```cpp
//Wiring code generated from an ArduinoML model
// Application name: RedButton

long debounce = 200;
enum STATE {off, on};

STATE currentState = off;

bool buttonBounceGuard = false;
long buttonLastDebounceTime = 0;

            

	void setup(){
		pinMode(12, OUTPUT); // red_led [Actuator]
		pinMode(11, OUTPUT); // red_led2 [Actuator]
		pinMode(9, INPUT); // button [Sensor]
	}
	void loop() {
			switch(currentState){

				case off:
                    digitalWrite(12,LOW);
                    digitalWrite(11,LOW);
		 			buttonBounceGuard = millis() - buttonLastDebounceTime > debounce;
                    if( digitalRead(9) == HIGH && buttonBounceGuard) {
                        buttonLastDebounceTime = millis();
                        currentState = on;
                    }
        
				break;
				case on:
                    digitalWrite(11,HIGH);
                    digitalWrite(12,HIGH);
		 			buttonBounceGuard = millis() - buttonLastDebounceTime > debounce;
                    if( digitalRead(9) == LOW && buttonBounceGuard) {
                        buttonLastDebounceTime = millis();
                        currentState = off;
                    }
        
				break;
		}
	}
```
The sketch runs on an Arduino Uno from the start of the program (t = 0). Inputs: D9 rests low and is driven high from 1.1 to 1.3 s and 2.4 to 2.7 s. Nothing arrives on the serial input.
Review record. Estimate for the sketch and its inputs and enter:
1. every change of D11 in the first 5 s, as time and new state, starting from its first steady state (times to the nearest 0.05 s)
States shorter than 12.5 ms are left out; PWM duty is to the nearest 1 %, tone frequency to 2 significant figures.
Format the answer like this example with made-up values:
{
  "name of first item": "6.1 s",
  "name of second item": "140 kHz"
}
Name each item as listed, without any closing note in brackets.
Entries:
{
  "every change of D11 in the first 5 s, as time and new state, starting from its first steady state": "0 s low; 1.1 s high; 1.3 s low; 2.4 s high; 2.7 s low"
}
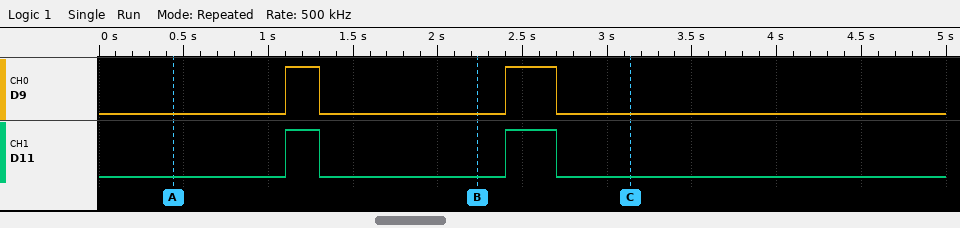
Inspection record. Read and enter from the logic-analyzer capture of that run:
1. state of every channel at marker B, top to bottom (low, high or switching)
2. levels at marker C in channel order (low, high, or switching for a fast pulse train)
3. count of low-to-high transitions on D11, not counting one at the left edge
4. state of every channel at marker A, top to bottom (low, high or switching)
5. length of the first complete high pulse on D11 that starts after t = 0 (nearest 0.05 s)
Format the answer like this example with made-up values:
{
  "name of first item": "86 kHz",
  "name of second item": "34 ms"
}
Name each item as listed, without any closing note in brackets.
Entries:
{
  "state of every channel at marker B, top to bottom": "D9 low, D11 low",
  "levels at marker C in channel order": "D9 low, D11 low",
  "count of low-to-high transitions on D11, not counting one at the left edge": "2",
  "state of every channel at marker A, top to bottom": "D9 low, D11 low",
  "length of the first complete high pulse on D11 that starts after t = 0": "0.20 s"
}
